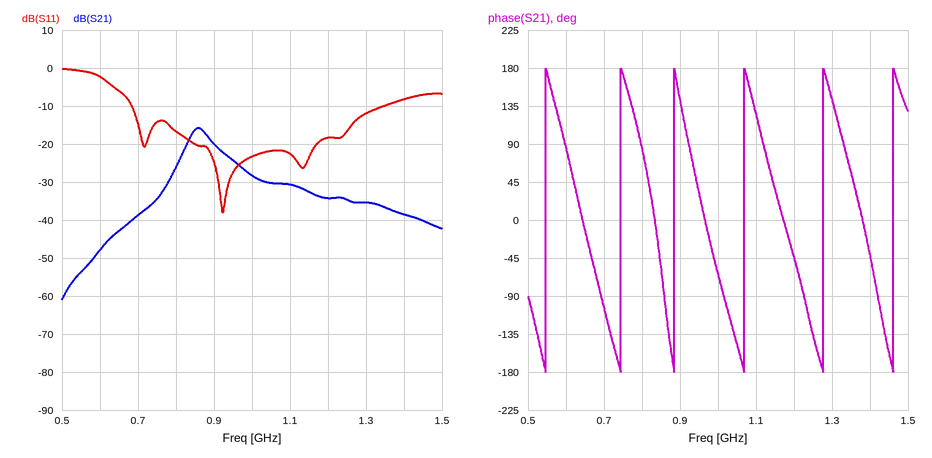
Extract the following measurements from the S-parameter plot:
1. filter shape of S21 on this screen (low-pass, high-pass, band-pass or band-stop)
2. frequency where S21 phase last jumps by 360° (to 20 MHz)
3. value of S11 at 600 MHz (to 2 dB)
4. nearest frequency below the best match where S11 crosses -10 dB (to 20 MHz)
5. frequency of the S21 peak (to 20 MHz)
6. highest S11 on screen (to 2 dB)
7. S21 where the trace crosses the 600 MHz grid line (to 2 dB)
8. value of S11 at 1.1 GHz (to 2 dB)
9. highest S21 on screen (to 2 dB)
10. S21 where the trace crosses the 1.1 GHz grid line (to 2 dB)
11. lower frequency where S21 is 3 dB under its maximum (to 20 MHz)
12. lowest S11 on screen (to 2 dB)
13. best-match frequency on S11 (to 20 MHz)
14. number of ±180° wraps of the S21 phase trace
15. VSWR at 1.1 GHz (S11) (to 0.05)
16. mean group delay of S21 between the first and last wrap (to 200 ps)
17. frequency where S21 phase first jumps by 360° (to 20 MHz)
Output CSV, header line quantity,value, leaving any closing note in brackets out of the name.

quantity,value
filter shape of S21 on this screen,band-pass
frequency where S21 phase last jumps by 360°,1.46 GHz
value of S11 at 600 MHz,-2 dB
nearest frequency below the best match where S11 crosses -10 dB,680 MHz
frequency of the S21 peak,860 MHz
highest S11 on screen,0 dB
S21 where the trace crosses the 600 MHz grid line,-48 dB
value of S11 at 1.1 GHz,-22 dB
highest S21 on screen,-16 dB
S21 where the trace crosses the 1.1 GHz grid line,-30 dB
lower frequency where S21 is 3 dB under its maximum,840 MHz
lowest S11 on screen,-38 dB
best-match frequency on S11,920 MHz
number of ±180° wraps of the S21 phase trace,6
VSWR at 1.1 GHz (S11),1.15
mean group delay of S21 between the first and last wrap,5.4 ns
frequency where S21 phase first jumps by 360°,540 MHz
